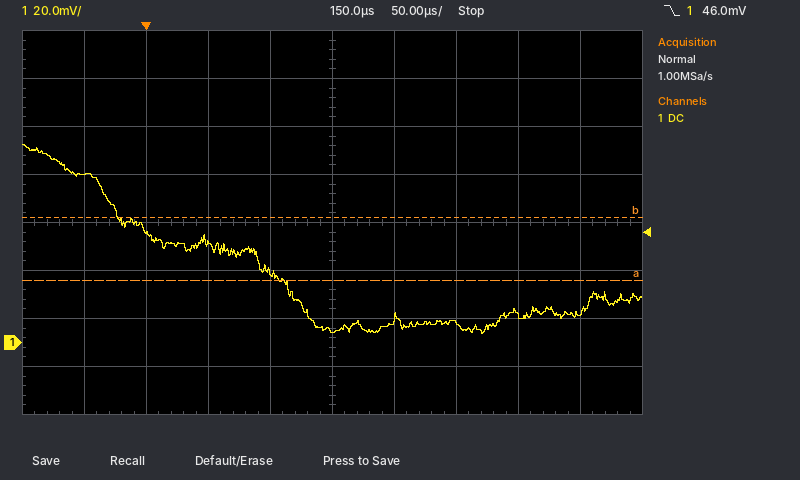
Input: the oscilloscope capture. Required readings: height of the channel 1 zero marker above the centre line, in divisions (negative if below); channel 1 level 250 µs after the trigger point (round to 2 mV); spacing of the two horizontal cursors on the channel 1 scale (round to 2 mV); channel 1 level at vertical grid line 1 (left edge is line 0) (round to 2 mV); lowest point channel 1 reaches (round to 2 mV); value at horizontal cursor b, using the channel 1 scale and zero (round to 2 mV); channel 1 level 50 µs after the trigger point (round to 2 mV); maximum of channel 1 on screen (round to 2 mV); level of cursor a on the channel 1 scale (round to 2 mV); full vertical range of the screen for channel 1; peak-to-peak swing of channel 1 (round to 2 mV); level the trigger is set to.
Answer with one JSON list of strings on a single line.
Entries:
["-2.5 div", "8 mV", "26 mV", "70 mV", "4 mV", "52 mV", "42 mV", "82 mV", "26 mV", "160 mV", "78 mV", "46.0 mV"]
